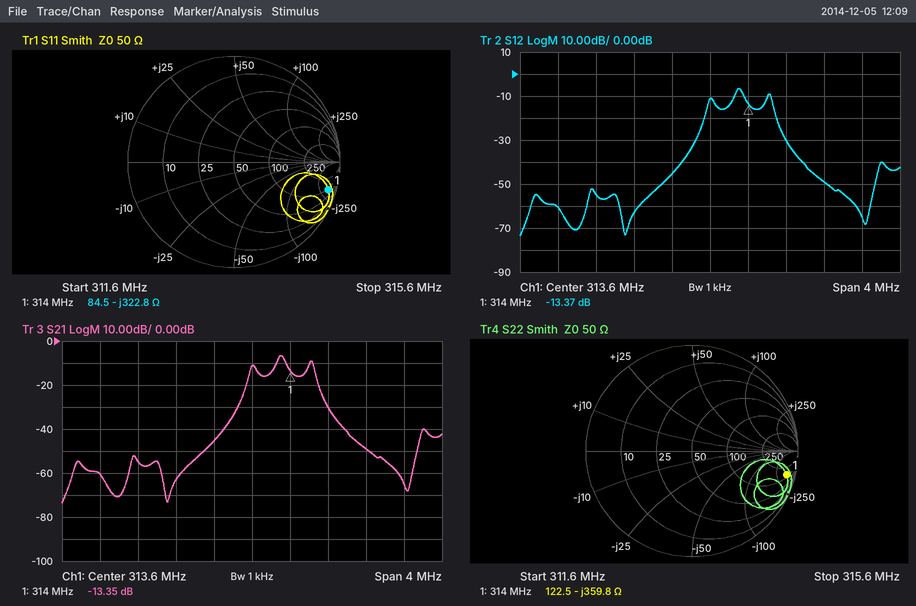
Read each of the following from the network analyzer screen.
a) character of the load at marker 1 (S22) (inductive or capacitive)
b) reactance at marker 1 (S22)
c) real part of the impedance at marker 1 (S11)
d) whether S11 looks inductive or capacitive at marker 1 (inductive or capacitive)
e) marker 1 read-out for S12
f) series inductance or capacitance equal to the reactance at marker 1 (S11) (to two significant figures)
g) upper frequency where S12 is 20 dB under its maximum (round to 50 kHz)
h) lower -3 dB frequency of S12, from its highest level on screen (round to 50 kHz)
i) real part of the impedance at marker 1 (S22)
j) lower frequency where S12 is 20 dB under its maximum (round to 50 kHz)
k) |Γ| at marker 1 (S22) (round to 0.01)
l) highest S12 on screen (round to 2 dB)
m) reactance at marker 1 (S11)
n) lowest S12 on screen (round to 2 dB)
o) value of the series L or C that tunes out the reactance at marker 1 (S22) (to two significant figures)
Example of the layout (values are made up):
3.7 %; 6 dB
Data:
capacitive; -359.8 Ω; 84.5 Ω; capacitive; -13.37 dB; 1.6 pF; 314.35 MHz; 313.85 MHz; 122.5 Ω; 313.50 MHz; 0.92; -6 dB; -322.8 Ω; -74 dB; 180 nH
